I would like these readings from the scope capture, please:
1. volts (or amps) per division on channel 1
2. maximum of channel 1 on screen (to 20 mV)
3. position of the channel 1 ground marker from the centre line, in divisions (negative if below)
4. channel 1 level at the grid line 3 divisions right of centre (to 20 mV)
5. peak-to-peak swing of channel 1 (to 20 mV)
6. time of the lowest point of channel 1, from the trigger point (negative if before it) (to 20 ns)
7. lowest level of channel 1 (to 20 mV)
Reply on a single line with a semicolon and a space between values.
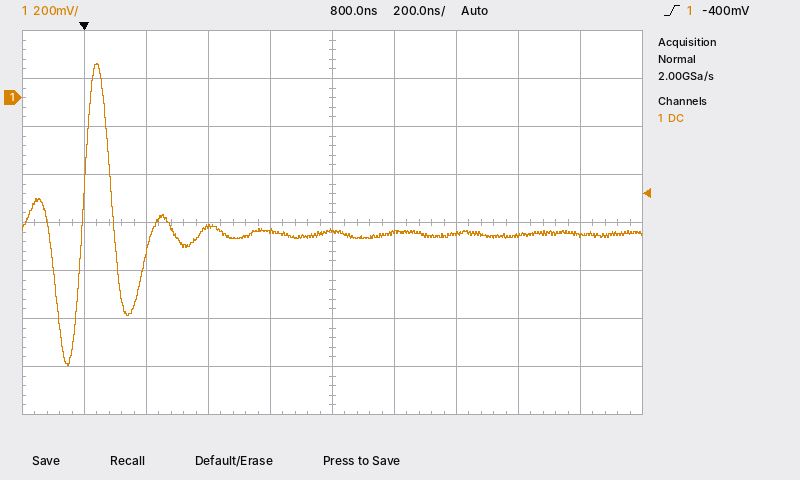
200 mV; 140 mV; +2.6 div; -580 mV; 1.26 V; -60 ns; -1.12 V
